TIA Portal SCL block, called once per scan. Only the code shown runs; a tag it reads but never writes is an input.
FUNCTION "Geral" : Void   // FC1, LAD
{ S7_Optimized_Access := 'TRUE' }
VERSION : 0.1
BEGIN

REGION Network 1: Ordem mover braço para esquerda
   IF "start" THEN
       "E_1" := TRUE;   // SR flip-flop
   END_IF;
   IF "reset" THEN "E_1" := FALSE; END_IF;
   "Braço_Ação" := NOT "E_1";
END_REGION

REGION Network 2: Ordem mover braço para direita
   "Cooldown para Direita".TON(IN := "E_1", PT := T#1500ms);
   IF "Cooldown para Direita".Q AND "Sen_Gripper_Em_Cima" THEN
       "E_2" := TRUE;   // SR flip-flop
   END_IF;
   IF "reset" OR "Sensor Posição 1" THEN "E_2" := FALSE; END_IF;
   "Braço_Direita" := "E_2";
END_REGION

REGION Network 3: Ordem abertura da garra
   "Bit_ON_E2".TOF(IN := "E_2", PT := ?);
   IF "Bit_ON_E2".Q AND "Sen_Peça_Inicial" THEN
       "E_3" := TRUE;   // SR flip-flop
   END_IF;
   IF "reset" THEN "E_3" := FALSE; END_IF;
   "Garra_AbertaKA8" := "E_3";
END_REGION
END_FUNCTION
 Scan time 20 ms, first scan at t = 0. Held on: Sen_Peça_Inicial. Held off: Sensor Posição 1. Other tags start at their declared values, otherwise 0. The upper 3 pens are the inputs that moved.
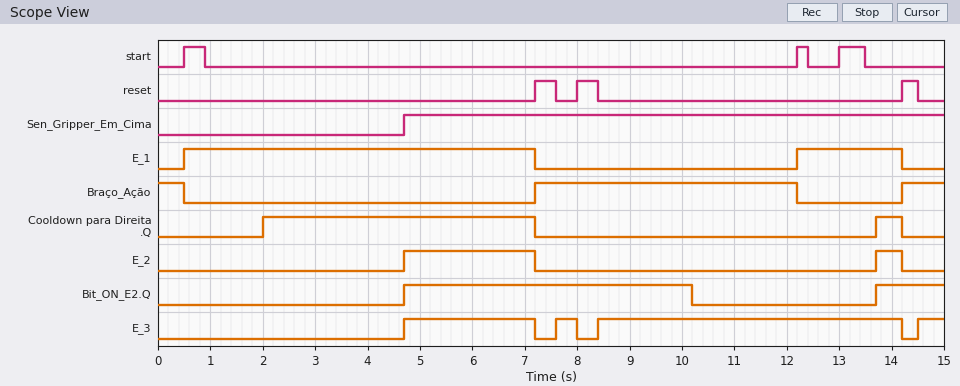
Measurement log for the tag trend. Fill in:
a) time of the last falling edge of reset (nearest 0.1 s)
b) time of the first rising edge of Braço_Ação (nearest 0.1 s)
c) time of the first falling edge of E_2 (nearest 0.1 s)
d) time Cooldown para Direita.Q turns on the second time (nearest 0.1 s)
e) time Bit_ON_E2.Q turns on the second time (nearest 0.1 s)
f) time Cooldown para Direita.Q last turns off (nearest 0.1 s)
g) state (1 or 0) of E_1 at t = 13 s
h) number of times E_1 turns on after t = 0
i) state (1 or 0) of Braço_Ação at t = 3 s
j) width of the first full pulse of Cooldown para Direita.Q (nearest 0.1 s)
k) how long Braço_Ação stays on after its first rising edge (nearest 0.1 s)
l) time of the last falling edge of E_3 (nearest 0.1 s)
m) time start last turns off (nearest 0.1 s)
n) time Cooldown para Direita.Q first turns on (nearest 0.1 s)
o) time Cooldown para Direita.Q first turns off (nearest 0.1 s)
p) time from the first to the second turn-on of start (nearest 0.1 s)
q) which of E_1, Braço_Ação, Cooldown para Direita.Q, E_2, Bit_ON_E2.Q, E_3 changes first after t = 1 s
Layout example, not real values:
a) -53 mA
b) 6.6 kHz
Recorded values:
a) 14.5 s
b) 7.2 s
c) 7.2 s
d) 13.7 s
e) 13.7 s
f) 14.2 s
g) 1
h) 2
i) 0
j) 5.2 s
k) 5.0 s
l) 14.2 s
m) 13.5 s
n) 2.0 s
o) 7.2 s
p) 11.7 s
q) Cooldown para Direita.Q
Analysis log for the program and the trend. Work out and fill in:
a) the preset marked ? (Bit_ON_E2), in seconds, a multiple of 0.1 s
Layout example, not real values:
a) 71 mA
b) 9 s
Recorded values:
a) 3.0 s
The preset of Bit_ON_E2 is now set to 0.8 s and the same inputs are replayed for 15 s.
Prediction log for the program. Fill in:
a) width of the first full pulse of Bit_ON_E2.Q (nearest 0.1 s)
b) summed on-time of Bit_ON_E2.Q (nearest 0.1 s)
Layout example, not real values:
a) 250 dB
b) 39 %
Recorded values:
a) 3.3 s
b) 4.6 s
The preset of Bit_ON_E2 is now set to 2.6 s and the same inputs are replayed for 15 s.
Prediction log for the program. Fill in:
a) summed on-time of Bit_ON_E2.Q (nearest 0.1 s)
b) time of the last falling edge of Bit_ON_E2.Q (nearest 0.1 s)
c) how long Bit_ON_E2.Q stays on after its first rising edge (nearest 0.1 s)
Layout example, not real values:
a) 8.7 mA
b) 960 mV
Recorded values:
a) 6.4 s
b) 9.8 s
c) 5.1 s
